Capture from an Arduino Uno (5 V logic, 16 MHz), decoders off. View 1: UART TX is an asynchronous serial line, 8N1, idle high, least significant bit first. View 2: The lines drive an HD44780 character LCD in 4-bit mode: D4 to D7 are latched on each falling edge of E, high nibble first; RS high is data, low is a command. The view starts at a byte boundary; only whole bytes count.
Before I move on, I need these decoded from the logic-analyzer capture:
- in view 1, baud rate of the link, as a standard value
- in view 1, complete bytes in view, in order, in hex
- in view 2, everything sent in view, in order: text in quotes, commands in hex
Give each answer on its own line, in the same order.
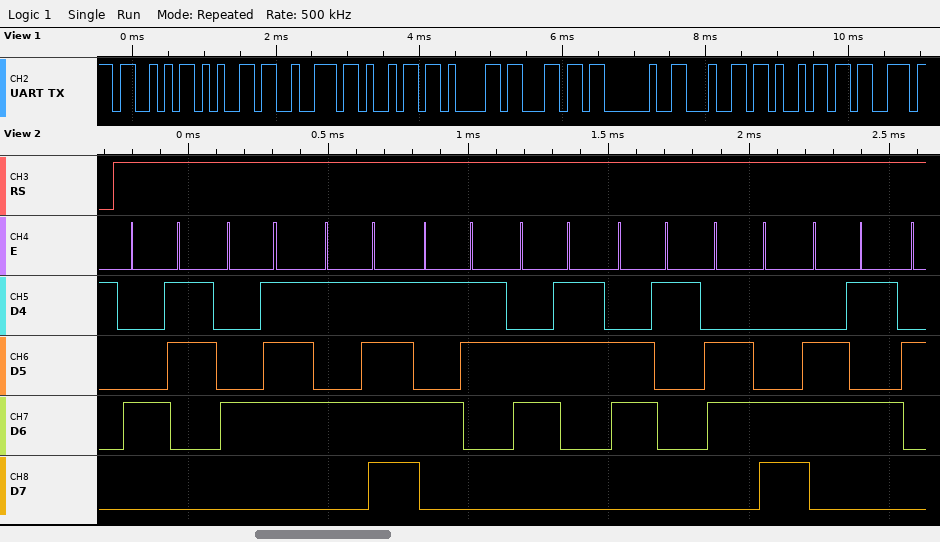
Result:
9600 baud
0x53 0x65 0x72 0x69 0x61 0x6C 0x20 0x64 0x69 0x73
"CG_Scale"
